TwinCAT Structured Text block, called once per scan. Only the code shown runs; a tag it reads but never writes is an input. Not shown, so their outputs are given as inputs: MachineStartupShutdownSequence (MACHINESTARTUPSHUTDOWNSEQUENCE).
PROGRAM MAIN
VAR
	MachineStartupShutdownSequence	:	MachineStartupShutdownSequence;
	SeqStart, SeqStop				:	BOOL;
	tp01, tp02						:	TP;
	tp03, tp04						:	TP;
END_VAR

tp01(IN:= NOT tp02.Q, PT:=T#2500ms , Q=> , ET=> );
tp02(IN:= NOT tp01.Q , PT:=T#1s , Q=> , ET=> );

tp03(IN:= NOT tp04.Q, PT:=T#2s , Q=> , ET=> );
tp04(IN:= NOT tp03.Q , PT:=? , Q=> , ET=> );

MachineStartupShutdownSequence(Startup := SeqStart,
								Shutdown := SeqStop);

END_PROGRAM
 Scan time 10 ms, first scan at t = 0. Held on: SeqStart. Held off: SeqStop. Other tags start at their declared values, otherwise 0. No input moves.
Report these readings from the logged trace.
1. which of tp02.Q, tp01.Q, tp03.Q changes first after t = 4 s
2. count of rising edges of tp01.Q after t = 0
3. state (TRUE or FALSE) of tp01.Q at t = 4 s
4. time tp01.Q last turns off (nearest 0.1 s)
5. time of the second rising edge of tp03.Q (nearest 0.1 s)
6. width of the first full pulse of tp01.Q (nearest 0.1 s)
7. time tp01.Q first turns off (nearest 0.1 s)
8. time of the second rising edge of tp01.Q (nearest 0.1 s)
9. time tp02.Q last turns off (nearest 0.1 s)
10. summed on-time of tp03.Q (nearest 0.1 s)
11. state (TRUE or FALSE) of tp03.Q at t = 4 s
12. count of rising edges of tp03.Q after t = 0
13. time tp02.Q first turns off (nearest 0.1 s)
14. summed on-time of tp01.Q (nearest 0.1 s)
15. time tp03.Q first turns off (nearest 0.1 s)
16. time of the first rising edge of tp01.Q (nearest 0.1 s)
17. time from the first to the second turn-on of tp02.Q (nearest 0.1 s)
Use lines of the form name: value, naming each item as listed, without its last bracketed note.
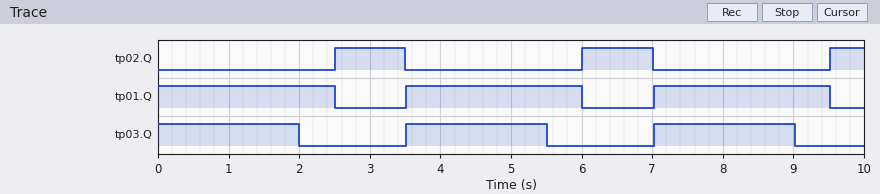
which of tp02.Q, tp01.Q, tp03.Q changes first after t = 4 s: tp03.Q
count of rising edges of tp01.Q after t = 0: 2
state (TRUE or FALSE) of tp01.Q at t = 4 s: TRUE
time tp01.Q last turns off: 9.5 s
time of the second rising edge of tp03.Q: 7.0 s
width of the first full pulse of tp01.Q: 2.5 s
time tp01.Q first turns off: 2.5 s
time of the second rising edge of tp01.Q: 7.0 s
time tp02.Q last turns off: 7.0 s
summed on-time of tp03.Q: 6.0 s
state (TRUE or FALSE) of tp03.Q at t = 4 s: TRUE
count of rising edges of tp03.Q after t = 0: 2
time tp02.Q first turns off: 3.5 s
summed on-time of tp01.Q: 7.5 s
time tp03.Q first turns off: 2.0 s
time of the first rising edge of tp01.Q: 3.5 s
time from the first to the second turn-on of tp02.Q: 3.5 s
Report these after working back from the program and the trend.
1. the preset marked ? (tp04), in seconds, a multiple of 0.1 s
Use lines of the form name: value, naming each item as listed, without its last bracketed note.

the preset marked ? (tp04), in seconds, a multiple of 0.1 s: 1.5 s
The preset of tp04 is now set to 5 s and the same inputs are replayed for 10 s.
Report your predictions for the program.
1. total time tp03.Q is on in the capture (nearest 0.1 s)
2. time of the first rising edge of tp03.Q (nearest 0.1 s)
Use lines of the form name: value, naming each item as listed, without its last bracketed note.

total time tp03.Q is on in the capture: 4.0 s
time of the first rising edge of tp03.Q: 7.0 s
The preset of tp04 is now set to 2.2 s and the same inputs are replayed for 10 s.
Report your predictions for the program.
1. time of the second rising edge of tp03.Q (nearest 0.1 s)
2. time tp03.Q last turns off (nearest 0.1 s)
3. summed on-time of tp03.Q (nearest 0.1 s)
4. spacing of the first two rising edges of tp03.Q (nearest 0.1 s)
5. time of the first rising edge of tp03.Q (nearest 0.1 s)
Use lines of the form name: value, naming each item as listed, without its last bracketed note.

time of the second rising edge of tp03.Q: 8.4 s
time tp03.Q last turns off: 6.2 s
summed on-time of tp03.Q: 5.6 s
spacing of the first two rising edges of tp03.Q: 4.2 s
time of the first rising edge of tp03.Q: 4.2 s
